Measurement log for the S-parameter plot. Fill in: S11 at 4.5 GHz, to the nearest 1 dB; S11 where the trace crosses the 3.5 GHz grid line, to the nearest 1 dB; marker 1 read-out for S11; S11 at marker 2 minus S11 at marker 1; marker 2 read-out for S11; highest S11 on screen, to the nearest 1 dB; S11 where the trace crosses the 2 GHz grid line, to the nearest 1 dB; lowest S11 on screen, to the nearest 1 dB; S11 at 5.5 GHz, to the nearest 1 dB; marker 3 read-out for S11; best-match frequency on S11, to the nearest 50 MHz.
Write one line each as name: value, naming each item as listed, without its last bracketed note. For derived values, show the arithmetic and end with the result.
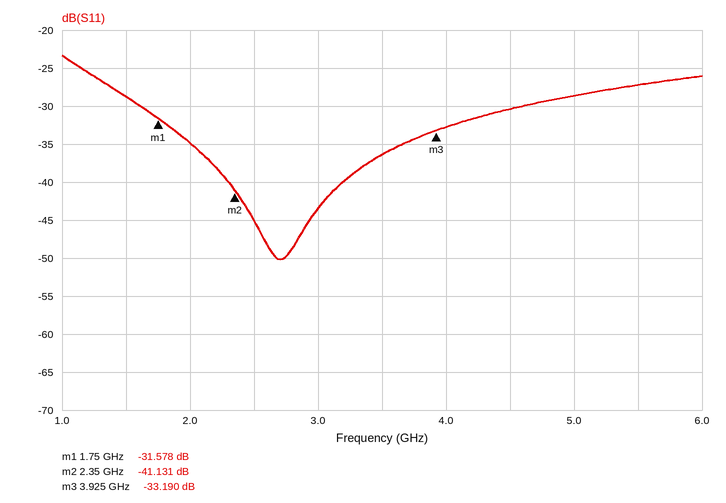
S11 at 4.5 GHz, to the nearest 1 dB: -30 dB
S11 where the trace crosses the 3.5 GHz grid line, to the nearest 1 dB: -36 dB
marker 1 read-out for S11: -31.578 dB
S11 at marker 2 minus S11 at marker 1: -41.131 − (-31.578) = -9.553 dB
marker 2 read-out for S11: -41.131 dB
highest S11 on screen, to the nearest 1 dB: -23 dB
S11 where the trace crosses the 2 GHz grid line, to the nearest 1 dB: -35 dB
lowest S11 on screen, to the nearest 1 dB: -50 dB
S11 at 5.5 GHz, to the nearest 1 dB: -27 dB
marker 3 read-out for S11: -33.190 dB
best-match frequency on S11, to the nearest 50 MHz: 2.70 GHz
